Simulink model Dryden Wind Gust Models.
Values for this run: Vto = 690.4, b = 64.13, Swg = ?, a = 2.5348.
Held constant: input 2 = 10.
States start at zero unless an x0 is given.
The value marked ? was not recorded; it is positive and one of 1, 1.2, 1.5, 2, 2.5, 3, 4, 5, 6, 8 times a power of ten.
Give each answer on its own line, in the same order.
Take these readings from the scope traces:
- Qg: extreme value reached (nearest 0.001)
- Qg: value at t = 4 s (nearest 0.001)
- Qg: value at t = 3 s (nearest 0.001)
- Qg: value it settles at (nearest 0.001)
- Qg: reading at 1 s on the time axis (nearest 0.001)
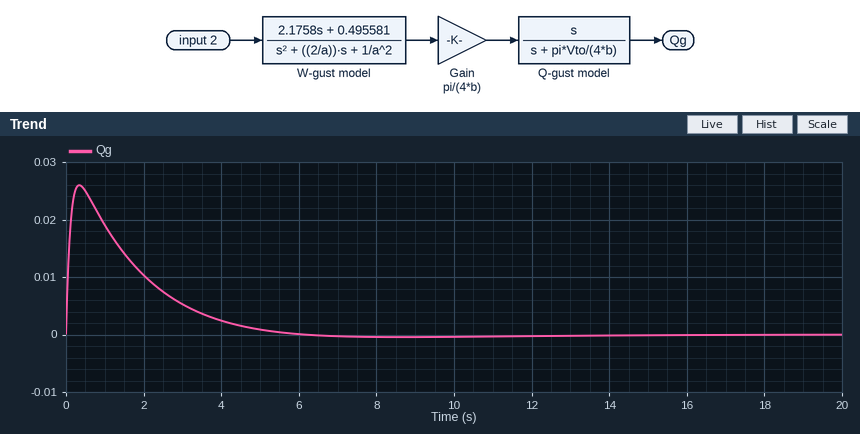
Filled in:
0.026
0.002
0.005
0.000
0.019
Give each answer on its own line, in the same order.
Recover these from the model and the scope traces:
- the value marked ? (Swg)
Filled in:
2
